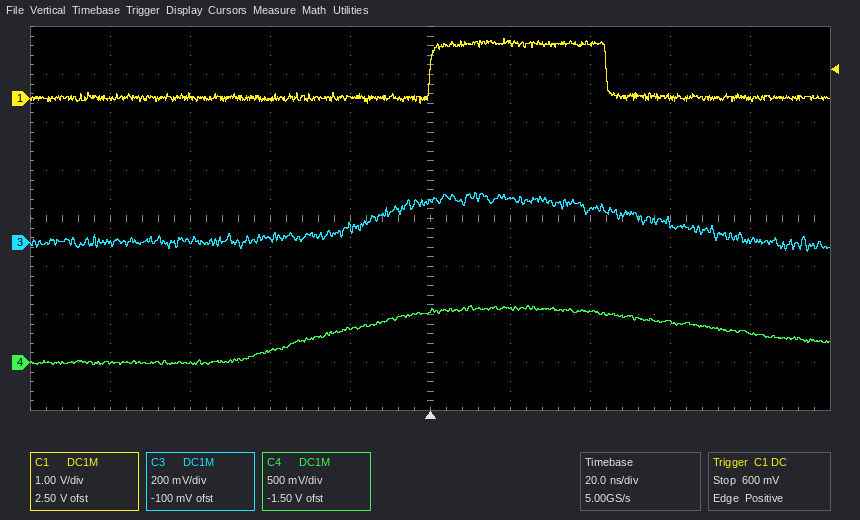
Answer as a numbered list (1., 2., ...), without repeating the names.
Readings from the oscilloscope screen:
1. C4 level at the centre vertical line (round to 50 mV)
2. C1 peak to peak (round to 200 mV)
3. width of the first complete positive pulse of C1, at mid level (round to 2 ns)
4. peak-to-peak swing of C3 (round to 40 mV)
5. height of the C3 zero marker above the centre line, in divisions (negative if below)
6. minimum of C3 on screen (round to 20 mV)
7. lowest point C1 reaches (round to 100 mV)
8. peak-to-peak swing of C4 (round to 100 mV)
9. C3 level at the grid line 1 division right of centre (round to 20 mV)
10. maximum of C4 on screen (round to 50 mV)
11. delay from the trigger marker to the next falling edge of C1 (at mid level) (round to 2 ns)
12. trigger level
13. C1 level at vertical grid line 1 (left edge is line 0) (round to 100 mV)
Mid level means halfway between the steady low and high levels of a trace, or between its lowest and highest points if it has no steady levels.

1. 550 mV
2. 1.4 V
3. 44 ns
4. 240 mV
5. -0.5 div
6. -40 mV
7. -100 mV
8. 600 mV
9. 180 mV
10. 600 mV
11. 44 ns
12. 600 mV
13. 0.0 V
